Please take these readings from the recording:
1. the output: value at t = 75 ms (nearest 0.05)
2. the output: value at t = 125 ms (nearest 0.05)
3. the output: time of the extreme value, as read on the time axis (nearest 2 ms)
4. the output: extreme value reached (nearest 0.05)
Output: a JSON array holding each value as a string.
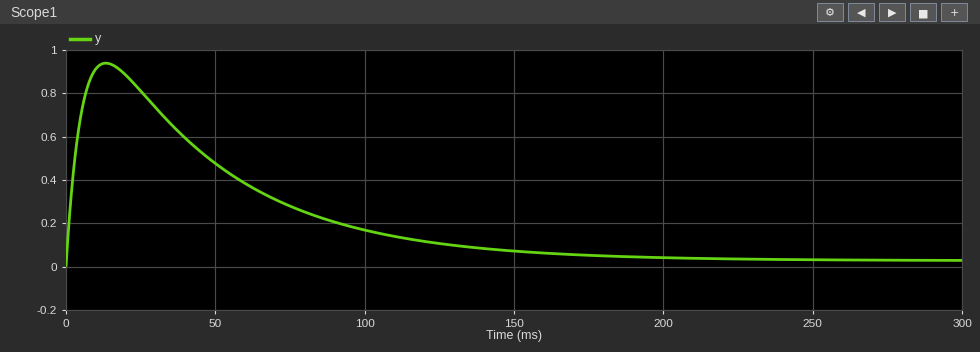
["0.30", "0.10", "14 ms", "0.95"]
